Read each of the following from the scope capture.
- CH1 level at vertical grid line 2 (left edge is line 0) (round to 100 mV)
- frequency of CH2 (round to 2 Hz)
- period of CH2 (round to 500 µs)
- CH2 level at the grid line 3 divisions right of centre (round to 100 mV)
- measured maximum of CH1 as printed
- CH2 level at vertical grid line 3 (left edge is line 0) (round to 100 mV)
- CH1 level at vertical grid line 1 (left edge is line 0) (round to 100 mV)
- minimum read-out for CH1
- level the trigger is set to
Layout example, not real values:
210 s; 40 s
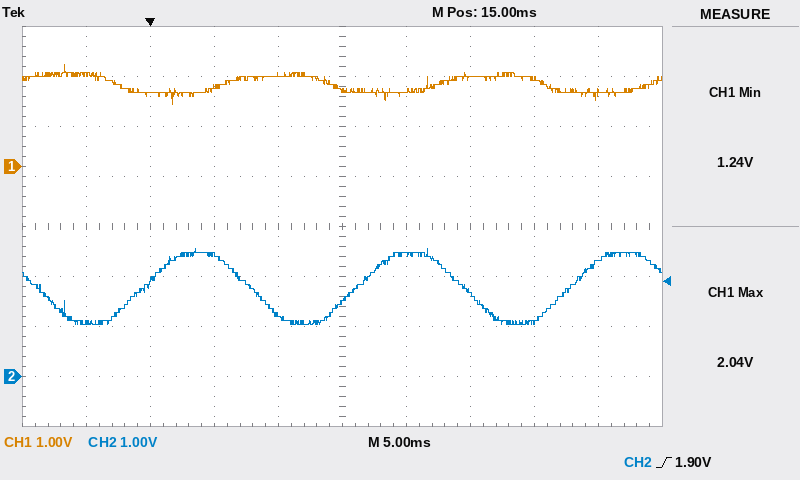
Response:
1.5 V; 60 Hz; 16.5 ms; 1.1 V; 2.04 V; 2.4 V; 1.8 V; 1.24 V; 1.90 V
